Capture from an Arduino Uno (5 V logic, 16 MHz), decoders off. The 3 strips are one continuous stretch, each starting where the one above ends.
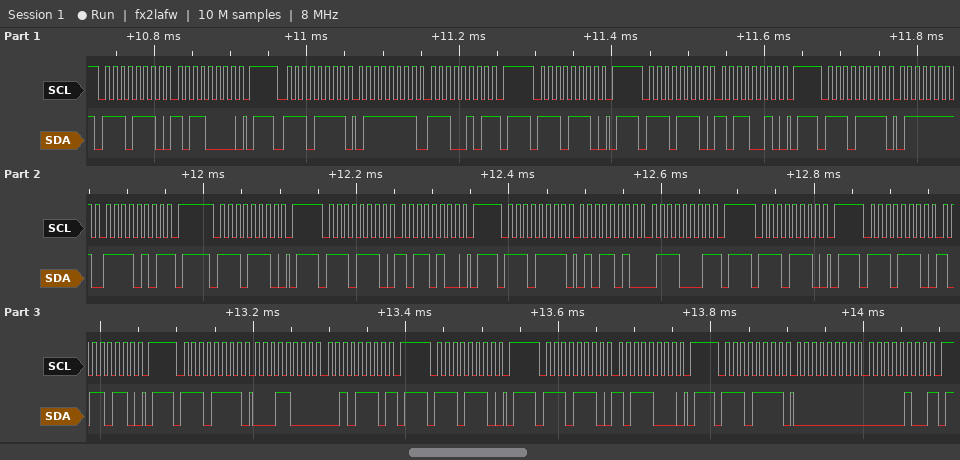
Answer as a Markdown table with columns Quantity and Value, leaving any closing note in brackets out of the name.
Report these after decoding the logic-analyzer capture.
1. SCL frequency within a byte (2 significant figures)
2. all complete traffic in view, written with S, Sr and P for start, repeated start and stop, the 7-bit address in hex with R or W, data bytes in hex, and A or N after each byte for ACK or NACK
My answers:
| Quantity | Value |
|---|---|
| SCL frequency within a byte | 100 kHz |
| all complete traffic in view, written with S, Sr and P for start, repeated start and stop, the 7-bit address in hex with R or W, data bytes in hex, and A or N after each byte for ACK or NACK | S 77W A B0 A P S 77R A 7F A E5 N P S 77W A P S 77W A B2 A P S 77R A 7F A F5 N P S 77W A P S 77W A B4 A P S 77R A 5A A 71 N P S 77W A P S 77W A B6 A P S 77R A 18 A 2E N P S 77W A P S 77W A B8 A P S 77R A 00 A 04 N P |
